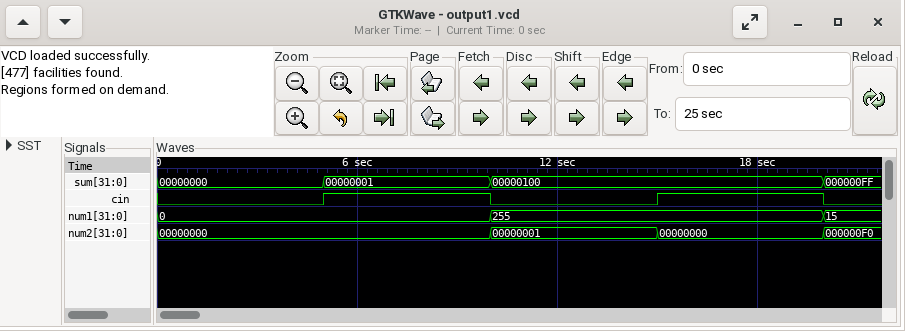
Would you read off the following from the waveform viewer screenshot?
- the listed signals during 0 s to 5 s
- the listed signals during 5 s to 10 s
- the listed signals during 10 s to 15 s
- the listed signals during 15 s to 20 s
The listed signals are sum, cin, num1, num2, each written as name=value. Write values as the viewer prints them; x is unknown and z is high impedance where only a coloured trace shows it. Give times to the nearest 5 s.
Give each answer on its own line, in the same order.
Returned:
sum=00000000, cin=0, num1=0, num2=00000000
sum=00000001, cin=1, num1=0, num2=00000000
sum=00000100, cin=0, num1=255, num2=00000001
sum=00000100, cin=1, num1=255, num2=00000000
